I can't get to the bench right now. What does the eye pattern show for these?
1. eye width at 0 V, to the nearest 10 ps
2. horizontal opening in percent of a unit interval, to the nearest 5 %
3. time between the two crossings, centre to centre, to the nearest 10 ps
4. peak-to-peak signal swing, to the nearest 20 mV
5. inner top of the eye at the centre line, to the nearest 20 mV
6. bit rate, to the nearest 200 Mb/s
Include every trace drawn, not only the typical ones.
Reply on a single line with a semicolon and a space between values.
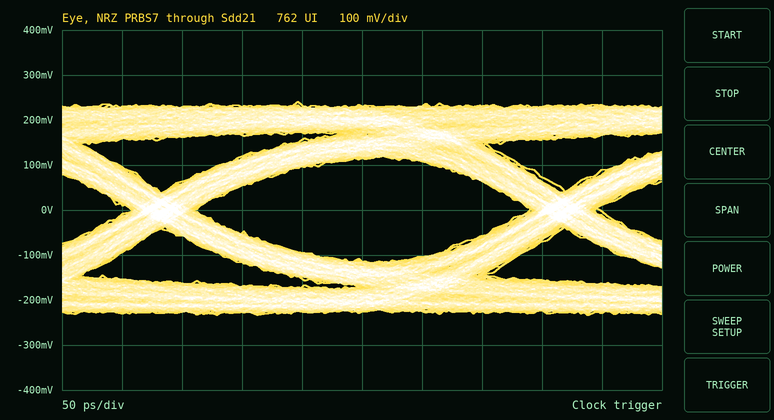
280 ps; 85 %; 330 ps; 480 mV; 120 mV; 3.0 Gb/s
